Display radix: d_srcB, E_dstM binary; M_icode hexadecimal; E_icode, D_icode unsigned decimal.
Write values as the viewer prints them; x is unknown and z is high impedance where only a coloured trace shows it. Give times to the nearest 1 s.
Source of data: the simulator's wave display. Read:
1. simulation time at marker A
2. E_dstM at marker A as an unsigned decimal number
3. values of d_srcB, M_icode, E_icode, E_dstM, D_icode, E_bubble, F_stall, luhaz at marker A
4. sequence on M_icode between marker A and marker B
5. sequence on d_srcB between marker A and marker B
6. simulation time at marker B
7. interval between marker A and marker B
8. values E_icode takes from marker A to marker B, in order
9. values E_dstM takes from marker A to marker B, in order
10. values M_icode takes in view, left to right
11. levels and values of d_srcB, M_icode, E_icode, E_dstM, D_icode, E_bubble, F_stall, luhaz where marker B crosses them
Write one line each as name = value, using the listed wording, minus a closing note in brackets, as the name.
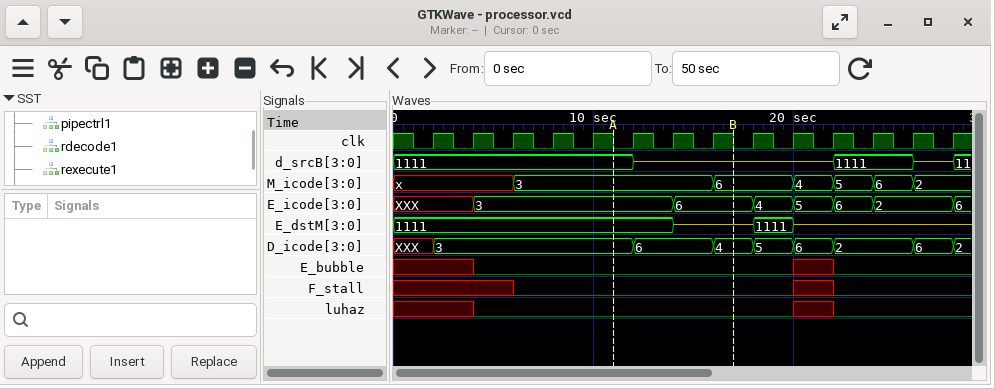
simulation time at marker A = 11 s
E_dstM at marker A as an unsigned decimal number = 15
values of d_srcB, M_icode, E_icode, E_dstM, D_icode, E_bubble, F_stall, luhaz at marker A = d_srcB=1111, M_icode=3, E_icode=3, E_dstM=1111, D_icode=3, E_bubble=0, F_stall=0, luhaz=0
sequence on M_icode between marker A and marker B = 3, 6
sequence on d_srcB between marker A and marker B = 1111, z
simulation time at marker B = 17 s
interval between marker A and marker B = 6 s
values E_icode takes from marker A to marker B, in order = 3, 6
values E_dstM takes from marker A to marker B, in order = 1111, z
values M_icode takes in view, left to right = x, 3, 6, 4, 5, 6, 2
levels and values of d_srcB, M_icode, E_icode, E_dstM, D_icode, E_bubble, F_stall, luhaz where marker B crosses them = d_srcB=z, M_icode=6, E_icode=6, E_dstM=z, D_icode=4, E_bubble=0, F_stall=0, luhaz=0
